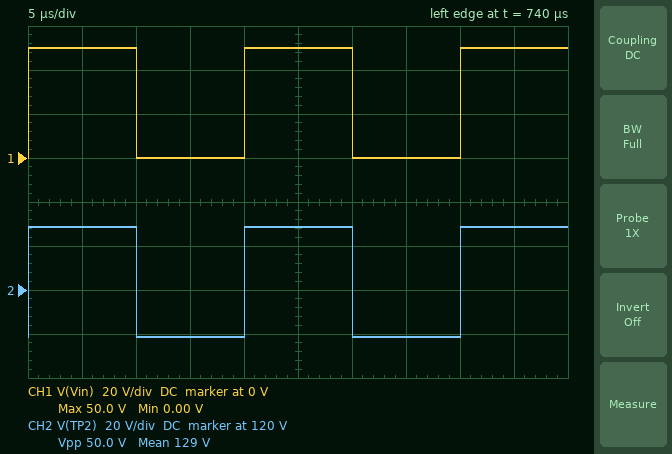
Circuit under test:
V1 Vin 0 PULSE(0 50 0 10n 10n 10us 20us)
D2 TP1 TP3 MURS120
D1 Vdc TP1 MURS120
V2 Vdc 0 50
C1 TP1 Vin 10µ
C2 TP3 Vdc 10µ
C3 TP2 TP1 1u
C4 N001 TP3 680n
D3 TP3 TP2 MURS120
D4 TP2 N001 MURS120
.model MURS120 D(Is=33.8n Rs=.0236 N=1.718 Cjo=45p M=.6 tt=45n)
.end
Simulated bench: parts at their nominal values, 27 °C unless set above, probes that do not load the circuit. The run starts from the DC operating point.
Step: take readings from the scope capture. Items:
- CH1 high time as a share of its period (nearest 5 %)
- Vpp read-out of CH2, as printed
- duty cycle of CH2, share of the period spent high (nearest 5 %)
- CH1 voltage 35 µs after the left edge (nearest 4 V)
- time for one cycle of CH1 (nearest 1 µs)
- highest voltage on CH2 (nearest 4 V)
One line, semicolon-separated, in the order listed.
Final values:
50 %; 50.0 V; 50 %; 0 V; 20 µs; 148 V
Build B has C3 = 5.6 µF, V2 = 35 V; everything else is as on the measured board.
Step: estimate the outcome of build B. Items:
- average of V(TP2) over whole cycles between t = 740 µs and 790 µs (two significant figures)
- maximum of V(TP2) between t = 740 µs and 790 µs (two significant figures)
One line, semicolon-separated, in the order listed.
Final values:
110 V; 130 V
